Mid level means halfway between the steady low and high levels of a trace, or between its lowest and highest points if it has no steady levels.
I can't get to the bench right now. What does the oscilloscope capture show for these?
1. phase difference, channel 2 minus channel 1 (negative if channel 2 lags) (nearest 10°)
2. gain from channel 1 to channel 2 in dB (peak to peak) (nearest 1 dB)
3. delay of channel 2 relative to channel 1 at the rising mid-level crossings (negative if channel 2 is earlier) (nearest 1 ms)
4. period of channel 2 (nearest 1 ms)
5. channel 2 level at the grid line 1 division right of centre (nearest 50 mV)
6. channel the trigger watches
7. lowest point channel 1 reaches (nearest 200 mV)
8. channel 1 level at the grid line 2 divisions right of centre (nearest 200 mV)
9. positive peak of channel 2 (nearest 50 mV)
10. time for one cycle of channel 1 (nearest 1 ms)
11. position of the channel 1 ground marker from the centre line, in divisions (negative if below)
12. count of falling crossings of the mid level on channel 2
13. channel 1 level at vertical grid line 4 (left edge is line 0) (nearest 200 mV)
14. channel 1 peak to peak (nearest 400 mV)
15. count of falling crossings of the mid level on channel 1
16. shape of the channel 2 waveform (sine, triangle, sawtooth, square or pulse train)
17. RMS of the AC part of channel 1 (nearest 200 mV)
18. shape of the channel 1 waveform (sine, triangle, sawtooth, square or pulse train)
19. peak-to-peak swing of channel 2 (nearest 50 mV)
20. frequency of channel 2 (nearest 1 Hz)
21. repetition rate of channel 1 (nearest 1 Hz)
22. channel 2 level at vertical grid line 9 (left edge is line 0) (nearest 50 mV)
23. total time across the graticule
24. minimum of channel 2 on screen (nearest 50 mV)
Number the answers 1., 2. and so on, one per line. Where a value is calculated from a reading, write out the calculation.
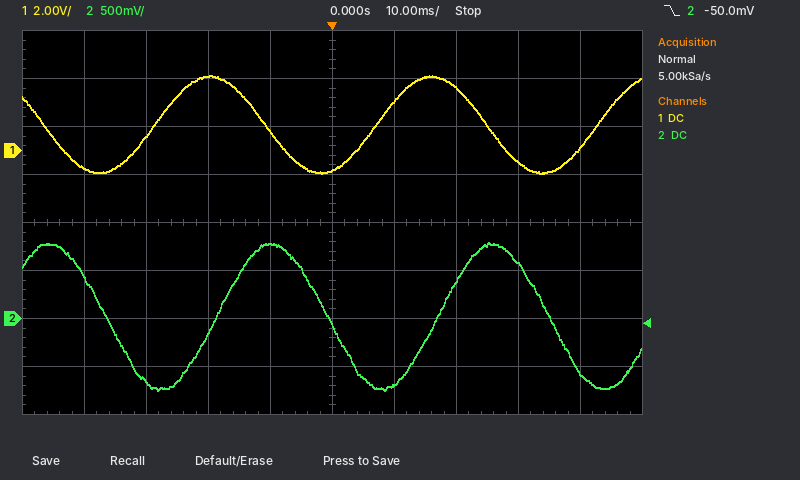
1. −360° × (+10 ms) / 36 ms ≈ -100°
2. 20 log10(1.55 V / 4.0 V) ≈ -8 dB
3. +10 ms
4. 36 ms
5. -700 mV
6. channel 2
7. -1.0 V
8. 2.6 V
9. 800 mV
10. 36 ms
11. +1.5 div
12. 3
13. 800 mV
14. 4.0 V
15. 3
16. sine
17. 4.0 V / (2√2) ≈ 1.4 V
18. sine
19. 800 mV − (-750 mV) = 1.55 V
20. 1 / 36 ms ≈ 28 Hz
21. 1 / 36 ms ≈ 28 Hz
22. -550 mV
23. 100 ms
24. -750 mV
